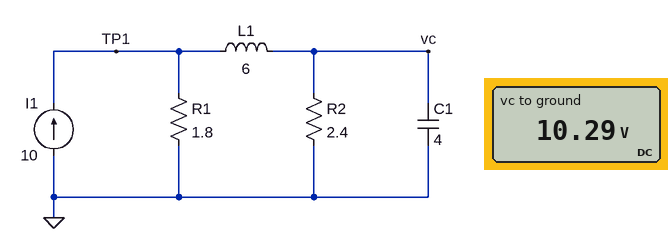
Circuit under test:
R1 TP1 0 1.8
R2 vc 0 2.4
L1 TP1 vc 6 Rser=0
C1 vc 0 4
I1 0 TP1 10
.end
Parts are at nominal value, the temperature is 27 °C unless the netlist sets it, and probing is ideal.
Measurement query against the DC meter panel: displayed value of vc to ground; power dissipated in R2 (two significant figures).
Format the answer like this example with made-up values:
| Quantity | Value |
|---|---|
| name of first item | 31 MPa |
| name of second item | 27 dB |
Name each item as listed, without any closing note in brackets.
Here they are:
| Quantity | Value |
|---|---|
| displayed value of vc to ground | 10.29 V |
| power dissipated in R2 | 44 W |
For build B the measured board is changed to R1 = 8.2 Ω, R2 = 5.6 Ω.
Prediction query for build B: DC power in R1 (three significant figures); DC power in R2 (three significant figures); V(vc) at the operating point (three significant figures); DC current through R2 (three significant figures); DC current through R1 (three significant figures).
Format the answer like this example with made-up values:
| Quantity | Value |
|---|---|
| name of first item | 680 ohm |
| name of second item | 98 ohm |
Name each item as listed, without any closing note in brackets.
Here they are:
| Quantity | Value |
|---|---|
| DC power in R1 | 135 W |
| DC power in R2 | 198 W |
| V(vc) at the operating point | 33.3 V |
| DC current through R2 | 5.94 A |
| DC current through R1 | 4.06 A |
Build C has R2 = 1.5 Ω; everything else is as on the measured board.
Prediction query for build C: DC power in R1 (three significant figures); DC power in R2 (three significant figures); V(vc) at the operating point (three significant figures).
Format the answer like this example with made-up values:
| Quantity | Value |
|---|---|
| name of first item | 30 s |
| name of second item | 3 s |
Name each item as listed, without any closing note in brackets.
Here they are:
| Quantity | Value |
|---|---|
| DC power in R1 | 37.2 W |
| DC power in R2 | 44.6 W |
| V(vc) at the operating point | 8.18 V |
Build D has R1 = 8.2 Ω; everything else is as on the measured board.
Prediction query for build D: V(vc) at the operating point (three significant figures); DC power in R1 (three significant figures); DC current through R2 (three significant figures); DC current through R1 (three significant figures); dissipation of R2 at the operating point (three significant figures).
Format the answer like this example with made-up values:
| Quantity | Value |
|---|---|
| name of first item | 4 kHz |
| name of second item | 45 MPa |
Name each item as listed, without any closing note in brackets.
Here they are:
| Quantity | Value |
|---|---|
| V(vc) at the operating point | 18.6 V |
| DC power in R1 | 42.0 W |
| DC current through R2 | 7.74 A |
| DC current through R1 | 2.26 A |
| dissipation of R2 at the operating point | 144 W |
